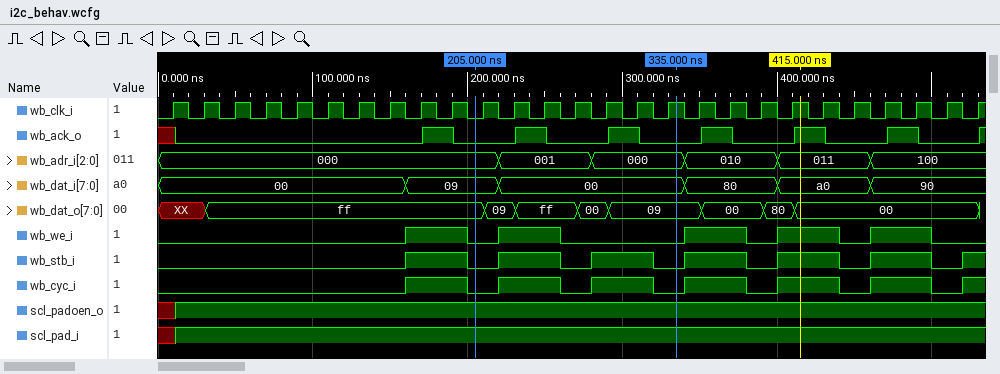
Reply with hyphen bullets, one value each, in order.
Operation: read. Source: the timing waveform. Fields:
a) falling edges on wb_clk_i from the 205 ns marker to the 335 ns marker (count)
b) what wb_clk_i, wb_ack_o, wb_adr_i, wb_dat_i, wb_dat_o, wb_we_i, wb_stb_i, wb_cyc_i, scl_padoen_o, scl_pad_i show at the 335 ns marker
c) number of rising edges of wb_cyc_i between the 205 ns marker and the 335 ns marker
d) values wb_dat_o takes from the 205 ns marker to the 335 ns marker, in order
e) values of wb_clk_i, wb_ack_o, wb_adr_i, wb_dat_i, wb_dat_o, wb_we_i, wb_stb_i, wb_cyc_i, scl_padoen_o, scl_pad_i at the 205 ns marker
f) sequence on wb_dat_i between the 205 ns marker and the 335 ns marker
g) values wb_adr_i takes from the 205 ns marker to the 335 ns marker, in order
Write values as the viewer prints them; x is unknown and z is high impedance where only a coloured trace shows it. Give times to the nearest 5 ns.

- 6
- wb_clk_i=1, wb_ack_o=0, wb_adr_i=000, wb_dat_i=00, wb_dat_o=09, wb_we_i=0, wb_stb_i=0, wb_cyc_i=0, scl_padoen_o=1, scl_pad_i=1
- 2
- ff, 09, ff, 00, 09
- wb_clk_i=0, wb_ack_o=0, wb_adr_i=000, wb_dat_i=09, wb_dat_o=ff, wb_we_i=0, wb_stb_i=0, wb_cyc_i=0, scl_padoen_o=1, scl_pad_i=1
- 09, 00
- 000, 001, 000
